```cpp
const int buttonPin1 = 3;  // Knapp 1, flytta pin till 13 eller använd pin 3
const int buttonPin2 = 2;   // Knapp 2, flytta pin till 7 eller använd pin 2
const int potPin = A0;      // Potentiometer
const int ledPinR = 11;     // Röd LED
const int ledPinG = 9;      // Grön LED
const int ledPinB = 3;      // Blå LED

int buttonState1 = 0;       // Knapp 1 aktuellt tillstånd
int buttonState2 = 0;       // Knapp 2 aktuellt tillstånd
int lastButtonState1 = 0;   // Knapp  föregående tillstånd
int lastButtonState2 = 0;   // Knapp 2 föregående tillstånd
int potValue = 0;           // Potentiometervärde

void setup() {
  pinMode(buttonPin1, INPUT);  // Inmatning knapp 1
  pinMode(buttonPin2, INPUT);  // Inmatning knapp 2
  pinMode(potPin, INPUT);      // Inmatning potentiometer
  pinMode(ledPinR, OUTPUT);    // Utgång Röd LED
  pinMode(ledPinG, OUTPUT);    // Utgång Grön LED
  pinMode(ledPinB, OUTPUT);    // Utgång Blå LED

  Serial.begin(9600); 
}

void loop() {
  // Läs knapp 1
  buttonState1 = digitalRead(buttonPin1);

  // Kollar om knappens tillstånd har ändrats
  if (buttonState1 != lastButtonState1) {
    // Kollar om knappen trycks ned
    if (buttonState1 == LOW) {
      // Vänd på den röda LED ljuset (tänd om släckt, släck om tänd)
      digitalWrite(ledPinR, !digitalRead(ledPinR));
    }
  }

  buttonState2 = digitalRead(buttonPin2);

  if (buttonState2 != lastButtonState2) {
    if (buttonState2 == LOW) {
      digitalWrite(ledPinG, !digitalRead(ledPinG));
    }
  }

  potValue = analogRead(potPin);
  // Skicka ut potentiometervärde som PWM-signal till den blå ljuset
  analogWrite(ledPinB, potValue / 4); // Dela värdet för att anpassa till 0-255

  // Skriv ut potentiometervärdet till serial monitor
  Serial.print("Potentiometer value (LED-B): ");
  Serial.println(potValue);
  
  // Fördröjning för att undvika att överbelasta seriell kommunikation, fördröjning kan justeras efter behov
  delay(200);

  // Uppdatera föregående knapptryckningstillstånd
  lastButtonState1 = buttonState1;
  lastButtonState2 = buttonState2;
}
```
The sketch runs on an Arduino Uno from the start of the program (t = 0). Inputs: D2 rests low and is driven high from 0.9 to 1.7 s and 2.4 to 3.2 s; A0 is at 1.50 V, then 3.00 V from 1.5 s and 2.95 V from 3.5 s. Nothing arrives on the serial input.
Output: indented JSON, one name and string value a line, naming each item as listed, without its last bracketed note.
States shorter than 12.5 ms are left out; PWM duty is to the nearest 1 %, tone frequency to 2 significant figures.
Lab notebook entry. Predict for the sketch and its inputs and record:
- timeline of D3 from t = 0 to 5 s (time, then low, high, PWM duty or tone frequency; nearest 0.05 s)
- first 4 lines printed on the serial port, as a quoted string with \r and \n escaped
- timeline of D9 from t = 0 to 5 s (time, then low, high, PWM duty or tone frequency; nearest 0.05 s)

{
  "timeline of D3 from t = 0 to 5 s": "0 s PWM 30 %; 1.6 s PWM 60 %; 3.6 s PWM 59 %",
  "first 4 lines printed on the serial port, as a quoted string with \\r and \\n escaped": "\"Potentiometer value (LED-B): 307\\r\\nPotentiometer value (LED-B): 307\\r\\nPotentiometer value (LED-B): 307\\r\\nPotentiometer value (LED-B): 307\\r\\n\"",
  "timeline of D9 from t = 0 to 5 s": "0 s low; 1.8 s high; 3.2 s low"
}
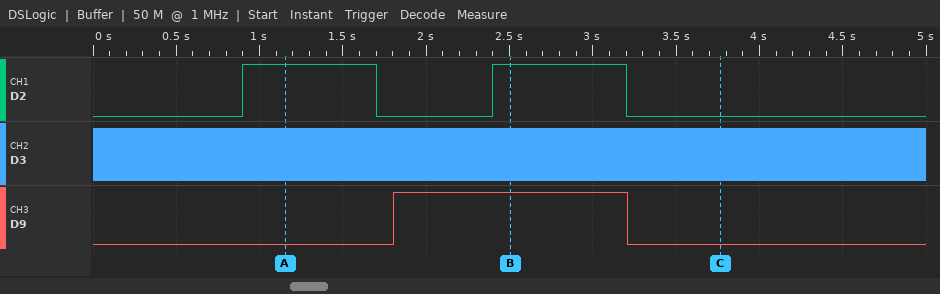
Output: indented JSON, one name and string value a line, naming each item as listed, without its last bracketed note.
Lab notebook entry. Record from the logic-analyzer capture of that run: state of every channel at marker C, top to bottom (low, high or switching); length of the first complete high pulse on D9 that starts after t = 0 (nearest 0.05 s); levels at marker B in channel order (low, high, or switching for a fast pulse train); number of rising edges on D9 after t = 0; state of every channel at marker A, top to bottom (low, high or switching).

{
  "state of every channel at marker C, top to bottom": "D2 low, D3 switching, D9 low",
  "length of the first complete high pulse on D9 that starts after t = 0": "1.40 s",
  "levels at marker B in channel order": "D2 high, D3 switching, D9 high",
  "number of rising edges on D9 after t = 0": "1",
  "state of every channel at marker A, top to bottom": "D2 high, D3 switching, D9 low"
}
